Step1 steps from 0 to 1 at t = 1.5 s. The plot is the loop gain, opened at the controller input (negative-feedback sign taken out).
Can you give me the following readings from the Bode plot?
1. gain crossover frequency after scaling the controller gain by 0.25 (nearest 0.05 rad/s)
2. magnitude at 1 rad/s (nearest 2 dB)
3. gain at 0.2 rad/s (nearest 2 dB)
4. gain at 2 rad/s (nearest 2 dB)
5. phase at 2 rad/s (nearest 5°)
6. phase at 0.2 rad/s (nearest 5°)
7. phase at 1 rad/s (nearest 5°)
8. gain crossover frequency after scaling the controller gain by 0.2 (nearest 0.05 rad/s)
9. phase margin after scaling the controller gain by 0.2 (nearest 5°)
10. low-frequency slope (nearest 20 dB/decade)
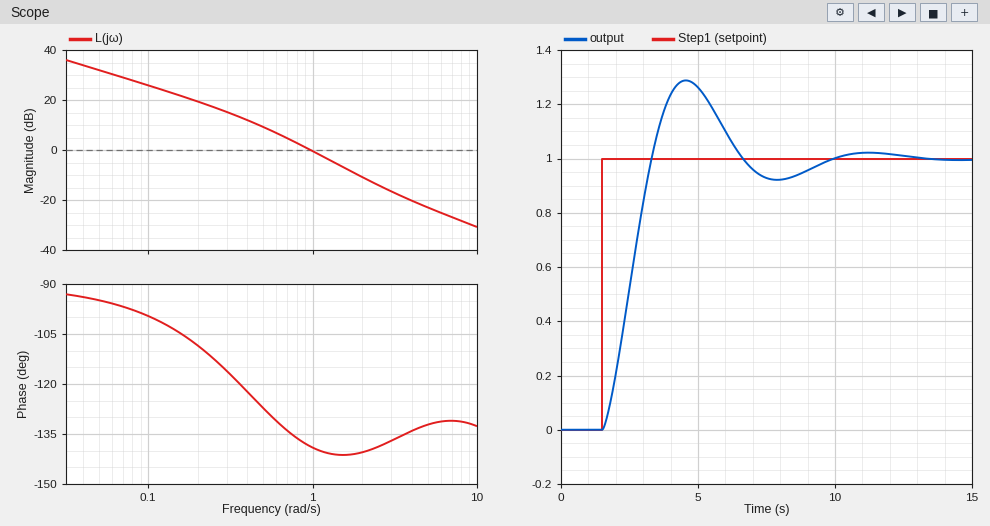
0.40 rad/s
0 dB
20 dB
-10 dB
-140°
-110°
-140°
0.35 rad/s
60°
-20 dB/decade
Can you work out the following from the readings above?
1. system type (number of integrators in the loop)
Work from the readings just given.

1
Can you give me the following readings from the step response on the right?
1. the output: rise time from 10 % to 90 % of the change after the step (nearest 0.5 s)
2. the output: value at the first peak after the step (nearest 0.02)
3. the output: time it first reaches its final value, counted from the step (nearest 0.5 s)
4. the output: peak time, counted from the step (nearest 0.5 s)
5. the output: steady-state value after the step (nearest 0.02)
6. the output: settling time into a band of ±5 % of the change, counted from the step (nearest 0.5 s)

1.5 s
1.28
2.0 s
3.0 s
1.00
7.5 s
